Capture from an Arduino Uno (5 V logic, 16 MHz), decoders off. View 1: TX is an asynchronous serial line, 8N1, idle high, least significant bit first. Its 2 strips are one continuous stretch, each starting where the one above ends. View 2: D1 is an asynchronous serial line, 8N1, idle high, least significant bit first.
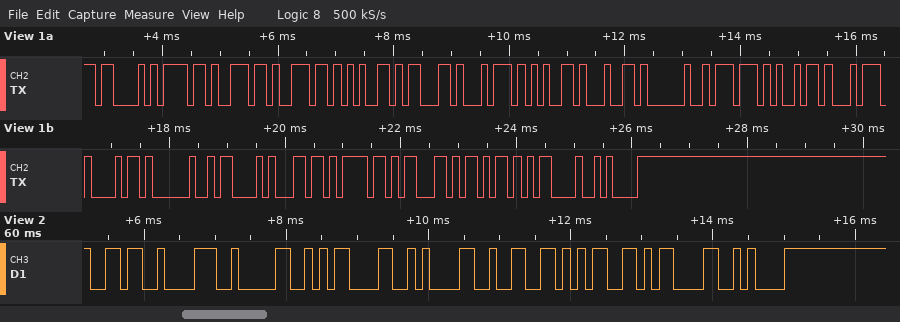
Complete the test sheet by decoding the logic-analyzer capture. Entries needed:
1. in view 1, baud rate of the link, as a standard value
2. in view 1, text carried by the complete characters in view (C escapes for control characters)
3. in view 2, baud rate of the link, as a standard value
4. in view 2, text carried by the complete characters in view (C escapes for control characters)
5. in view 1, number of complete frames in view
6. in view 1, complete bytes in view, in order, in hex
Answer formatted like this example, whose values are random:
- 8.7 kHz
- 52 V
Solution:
- 9600 baud
- "Connected with Clock\r\n"
- 9600 baud
- "680\r\n25\r\n"
- 22
- 43 6F 6E 6E 65 63 74 65 64 20 77 69 74 68 20 43 6C 6F 63 6B 0D 0A
